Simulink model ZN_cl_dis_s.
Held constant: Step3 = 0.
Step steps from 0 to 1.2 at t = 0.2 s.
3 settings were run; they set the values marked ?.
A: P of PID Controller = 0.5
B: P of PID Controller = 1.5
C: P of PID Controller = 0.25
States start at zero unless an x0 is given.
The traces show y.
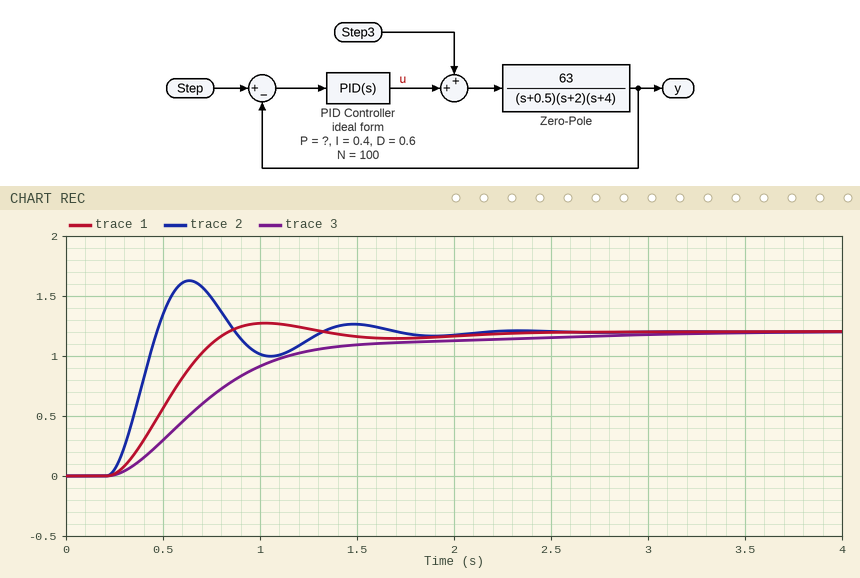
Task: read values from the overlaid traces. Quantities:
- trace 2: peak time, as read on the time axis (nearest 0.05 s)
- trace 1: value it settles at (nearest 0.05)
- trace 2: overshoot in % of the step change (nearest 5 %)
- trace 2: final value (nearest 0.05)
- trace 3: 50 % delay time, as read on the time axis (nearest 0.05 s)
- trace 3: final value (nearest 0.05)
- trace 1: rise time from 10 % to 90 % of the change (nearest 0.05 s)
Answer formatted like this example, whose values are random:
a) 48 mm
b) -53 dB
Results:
a) 0.65 s
b) 1.20
c) 35 %
d) 1.20
e) 0.70 s
f) 1.20
g) 0.40 s
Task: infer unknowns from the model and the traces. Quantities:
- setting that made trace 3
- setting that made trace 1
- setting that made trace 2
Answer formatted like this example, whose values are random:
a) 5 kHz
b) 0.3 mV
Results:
a) C
b) A
c) B
